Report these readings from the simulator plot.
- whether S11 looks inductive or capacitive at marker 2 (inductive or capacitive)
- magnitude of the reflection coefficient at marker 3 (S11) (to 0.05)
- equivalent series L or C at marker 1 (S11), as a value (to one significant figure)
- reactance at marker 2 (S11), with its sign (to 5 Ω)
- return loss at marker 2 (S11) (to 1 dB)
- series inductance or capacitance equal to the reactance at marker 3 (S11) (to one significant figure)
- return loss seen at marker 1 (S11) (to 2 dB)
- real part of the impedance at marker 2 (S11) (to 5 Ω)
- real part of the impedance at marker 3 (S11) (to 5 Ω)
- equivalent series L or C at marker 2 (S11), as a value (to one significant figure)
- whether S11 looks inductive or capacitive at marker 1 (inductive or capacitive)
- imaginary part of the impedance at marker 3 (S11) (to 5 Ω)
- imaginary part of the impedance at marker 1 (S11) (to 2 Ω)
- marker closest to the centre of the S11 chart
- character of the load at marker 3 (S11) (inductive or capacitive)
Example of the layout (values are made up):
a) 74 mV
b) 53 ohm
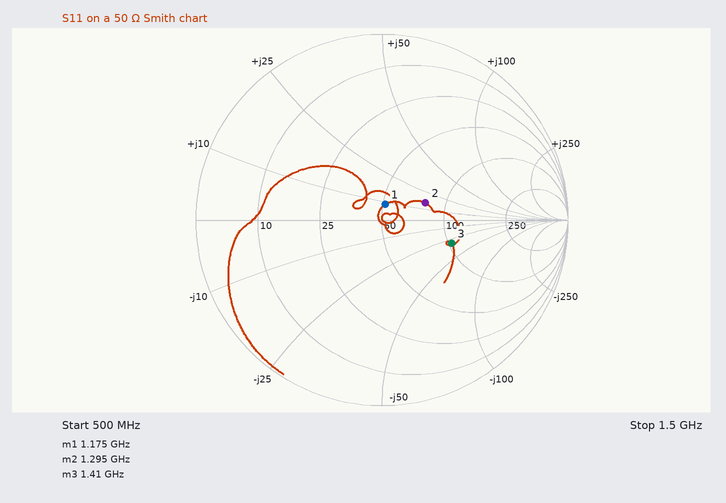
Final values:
a) inductive
b) 0.40
c) 1 nH
d) +15 Ω
e) 12 dB
f) 4 pF
g) 22 dB
h) 80 Ω
i) 105 Ω
j) 2 nH
k) inductive
l) -30 Ω
m) +8 Ω
n) marker 1
o) capacitive
